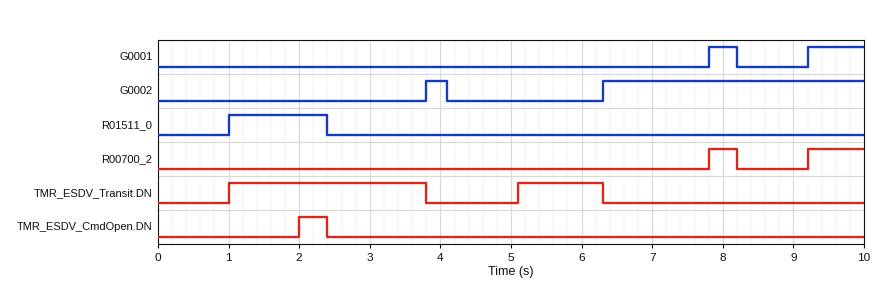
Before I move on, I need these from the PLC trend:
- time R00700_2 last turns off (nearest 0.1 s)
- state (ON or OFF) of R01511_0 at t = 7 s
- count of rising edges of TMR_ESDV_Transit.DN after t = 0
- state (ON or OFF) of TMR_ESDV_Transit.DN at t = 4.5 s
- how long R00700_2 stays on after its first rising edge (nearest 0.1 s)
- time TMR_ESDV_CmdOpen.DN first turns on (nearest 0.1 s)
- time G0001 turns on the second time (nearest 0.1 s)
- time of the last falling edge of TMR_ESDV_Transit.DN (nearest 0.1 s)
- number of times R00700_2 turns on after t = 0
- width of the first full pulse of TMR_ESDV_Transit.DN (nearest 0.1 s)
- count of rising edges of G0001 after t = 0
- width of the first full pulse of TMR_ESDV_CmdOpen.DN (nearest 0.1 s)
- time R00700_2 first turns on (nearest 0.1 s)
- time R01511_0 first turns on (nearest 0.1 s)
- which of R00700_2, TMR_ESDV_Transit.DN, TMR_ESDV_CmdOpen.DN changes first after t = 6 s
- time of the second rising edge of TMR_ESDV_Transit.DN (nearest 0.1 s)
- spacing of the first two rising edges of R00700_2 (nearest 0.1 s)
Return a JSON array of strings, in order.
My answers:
["8.2 s", "OFF", "2", "OFF", "0.4 s", "2.0 s", "9.2 s", "6.3 s", "2", "2.8 s", "2", "0.4 s", "7.8 s", "1.0 s", "TMR_ESDV_Transit.DN", "5.1 s", "1.4 s"]
